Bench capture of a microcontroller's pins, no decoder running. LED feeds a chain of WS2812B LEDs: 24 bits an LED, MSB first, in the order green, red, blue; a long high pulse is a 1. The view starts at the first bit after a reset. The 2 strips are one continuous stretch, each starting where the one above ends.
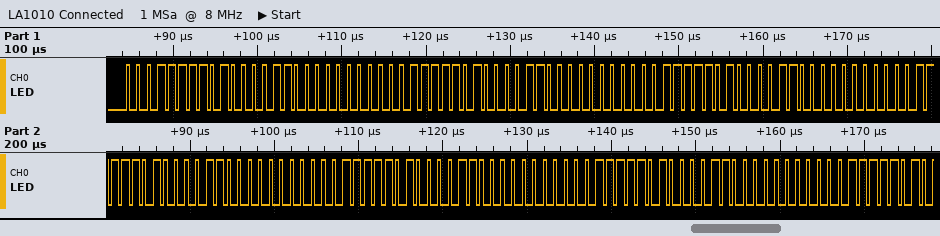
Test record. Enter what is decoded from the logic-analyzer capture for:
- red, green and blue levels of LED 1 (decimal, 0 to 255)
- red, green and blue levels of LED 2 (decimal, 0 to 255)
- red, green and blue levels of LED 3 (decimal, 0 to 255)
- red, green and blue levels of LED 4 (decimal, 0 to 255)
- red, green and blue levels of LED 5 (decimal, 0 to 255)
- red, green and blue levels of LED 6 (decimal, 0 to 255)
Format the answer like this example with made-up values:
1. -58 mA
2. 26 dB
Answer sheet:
1. 67, 31, 0
2. 67, 31, 0
3. 67, 31, 0
4. 67, 31, 0
5. 67, 31, 0
6. 67, 31, 0
